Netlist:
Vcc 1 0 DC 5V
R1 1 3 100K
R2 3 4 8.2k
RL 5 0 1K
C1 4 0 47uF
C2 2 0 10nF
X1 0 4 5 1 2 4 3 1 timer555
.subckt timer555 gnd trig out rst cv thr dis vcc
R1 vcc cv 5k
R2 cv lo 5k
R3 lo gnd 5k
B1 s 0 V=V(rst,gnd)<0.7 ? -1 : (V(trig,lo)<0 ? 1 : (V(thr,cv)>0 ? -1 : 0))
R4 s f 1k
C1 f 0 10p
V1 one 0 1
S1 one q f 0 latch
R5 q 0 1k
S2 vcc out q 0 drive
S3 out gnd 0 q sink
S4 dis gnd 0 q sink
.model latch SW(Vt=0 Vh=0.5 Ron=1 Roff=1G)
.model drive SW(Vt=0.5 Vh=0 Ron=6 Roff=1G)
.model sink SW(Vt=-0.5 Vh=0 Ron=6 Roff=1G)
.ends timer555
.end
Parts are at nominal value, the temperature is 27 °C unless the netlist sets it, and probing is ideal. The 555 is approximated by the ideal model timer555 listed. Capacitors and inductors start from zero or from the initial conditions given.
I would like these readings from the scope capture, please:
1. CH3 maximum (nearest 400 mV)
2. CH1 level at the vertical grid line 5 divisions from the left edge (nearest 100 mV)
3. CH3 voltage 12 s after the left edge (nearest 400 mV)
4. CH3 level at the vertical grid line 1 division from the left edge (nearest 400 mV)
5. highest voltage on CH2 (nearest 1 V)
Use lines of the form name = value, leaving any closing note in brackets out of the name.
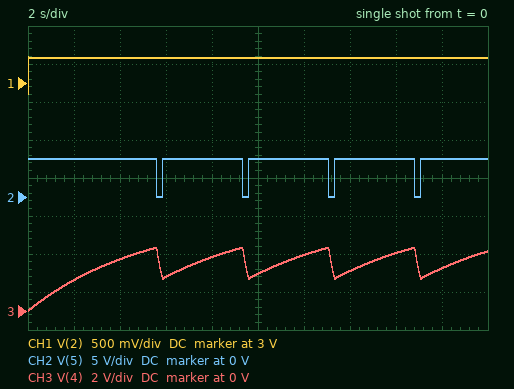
CH3 maximum = 3.2 V
CH1 level at the vertical grid line 5 divisions from the left edge = 3.3 V
CH3 voltage 12 s after the left edge = 2.8 V
CH3 level at the vertical grid line 1 division from the left edge = 1.6 V
highest voltage on CH2 = 5 V
